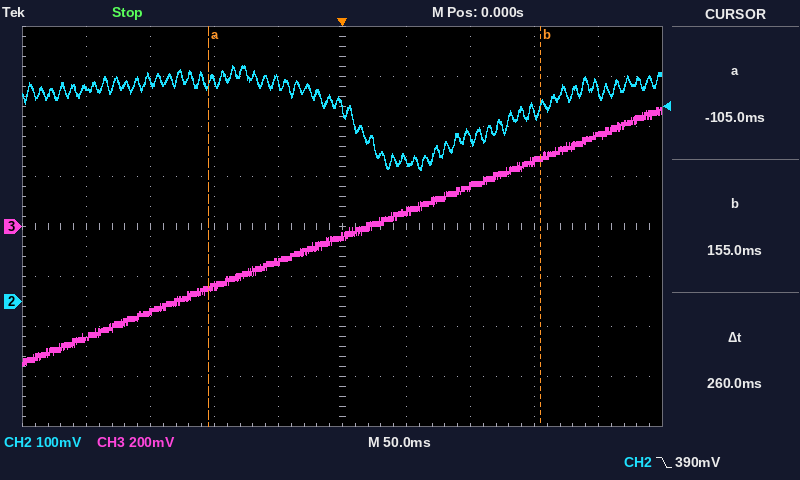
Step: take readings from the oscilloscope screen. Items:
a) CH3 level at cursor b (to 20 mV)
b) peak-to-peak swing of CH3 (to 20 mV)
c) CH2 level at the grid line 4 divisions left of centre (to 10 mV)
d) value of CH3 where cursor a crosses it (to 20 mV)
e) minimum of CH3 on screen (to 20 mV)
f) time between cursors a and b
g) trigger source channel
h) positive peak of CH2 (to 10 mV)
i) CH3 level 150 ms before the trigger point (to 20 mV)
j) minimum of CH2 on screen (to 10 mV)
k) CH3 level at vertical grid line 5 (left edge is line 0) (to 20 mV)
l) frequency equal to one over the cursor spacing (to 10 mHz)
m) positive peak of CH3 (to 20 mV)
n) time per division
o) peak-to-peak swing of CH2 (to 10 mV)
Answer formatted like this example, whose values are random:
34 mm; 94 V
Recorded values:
280 mV; 1.04 V; 430 mV; -240 mV; -560 mV; 260 ms; CH2; 470 mV; -340 mV; 260 mV; -40 mV; 3.85 Hz; 480 mV; 50 ms; 210 mV
